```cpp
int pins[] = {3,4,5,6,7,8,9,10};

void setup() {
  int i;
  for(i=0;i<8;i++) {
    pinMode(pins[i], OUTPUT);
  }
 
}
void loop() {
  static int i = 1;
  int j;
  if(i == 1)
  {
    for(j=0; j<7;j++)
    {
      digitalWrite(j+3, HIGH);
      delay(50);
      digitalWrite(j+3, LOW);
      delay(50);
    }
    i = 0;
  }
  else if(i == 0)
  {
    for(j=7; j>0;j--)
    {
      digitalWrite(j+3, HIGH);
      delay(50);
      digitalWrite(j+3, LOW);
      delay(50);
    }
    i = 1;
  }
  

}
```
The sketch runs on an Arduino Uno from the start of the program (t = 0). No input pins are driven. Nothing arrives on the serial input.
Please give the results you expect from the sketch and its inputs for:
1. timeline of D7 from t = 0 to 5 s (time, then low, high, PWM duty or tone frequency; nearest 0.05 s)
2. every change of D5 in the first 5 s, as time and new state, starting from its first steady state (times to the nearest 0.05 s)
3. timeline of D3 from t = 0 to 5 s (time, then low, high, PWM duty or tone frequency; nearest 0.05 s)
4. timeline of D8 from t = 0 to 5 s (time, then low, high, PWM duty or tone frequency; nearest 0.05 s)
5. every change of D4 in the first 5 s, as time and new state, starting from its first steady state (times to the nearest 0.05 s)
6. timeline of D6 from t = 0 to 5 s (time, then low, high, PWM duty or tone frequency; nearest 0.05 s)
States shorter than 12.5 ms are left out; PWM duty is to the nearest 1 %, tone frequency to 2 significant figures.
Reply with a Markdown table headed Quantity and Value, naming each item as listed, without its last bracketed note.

| Quantity | Value |
|---|---|
| timeline of D7 from t = 0 to 5 s | 0 s low; 0.4 s high; 0.45 s low; 1 s high; 1.05 s low; 1.8 s high; 1.85 s low; 2.4 s high; 2.45 s low; 3.2 s high; 3.25 s low; 3.8 s high; 3.85 s low; 4.6 s high; 4.65 s low |
| every change of D5 in the first 5 s, as time and new state, starting from its first steady state | 0 s low; 0.2 s high; 0.25 s low; 1.2 s high; 1.25 s low; 1.6 s high; 1.65 s low; 2.6 s high; 2.65 s low; 3 s high; 3.05 s low; 4 s high; 4.05 s low; 4.4 s high; 4.45 s low |
| timeline of D3 from t = 0 to 5 s | 0 s high; 0.05 s low; 1.4 s high; 1.45 s low; 2.8 s high; 2.85 s low; 4.2 s high; 4.25 s low |
| timeline of D8 from t = 0 to 5 s | 0 s low; 0.5 s high; 0.55 s low; 0.9 s high; 0.95 s low; 1.9 s high; 1.95 s low; 2.3 s high; 2.35 s low; 3.3 s high; 3.35 s low; 3.7 s high; 3.75 s low; 4.7 s high; 4.75 s low |
| every change of D4 in the first 5 s, as time and new state, starting from its first steady state | 0 s low; 0.1 s high; 0.15 s low; 1.3 s high; 1.35 s low; 1.5 s high; 1.55 s low; 2.7 s high; 2.75 s low; 2.9 s high; 2.95 s low; 4.1 s high; 4.15 s low; 4.3 s high; 4.35 s low |
| timeline of D6 from t = 0 to 5 s | 0 s low; 0.3 s high; 0.35 s low; 1.1 s high; 1.15 s low; 1.7 s high; 1.75 s low; 2.5 s high; 2.55 s low; 3.1 s high; 3.15 s low; 3.9 s high; 3.95 s low; 4.5 s high; 4.55 s low |
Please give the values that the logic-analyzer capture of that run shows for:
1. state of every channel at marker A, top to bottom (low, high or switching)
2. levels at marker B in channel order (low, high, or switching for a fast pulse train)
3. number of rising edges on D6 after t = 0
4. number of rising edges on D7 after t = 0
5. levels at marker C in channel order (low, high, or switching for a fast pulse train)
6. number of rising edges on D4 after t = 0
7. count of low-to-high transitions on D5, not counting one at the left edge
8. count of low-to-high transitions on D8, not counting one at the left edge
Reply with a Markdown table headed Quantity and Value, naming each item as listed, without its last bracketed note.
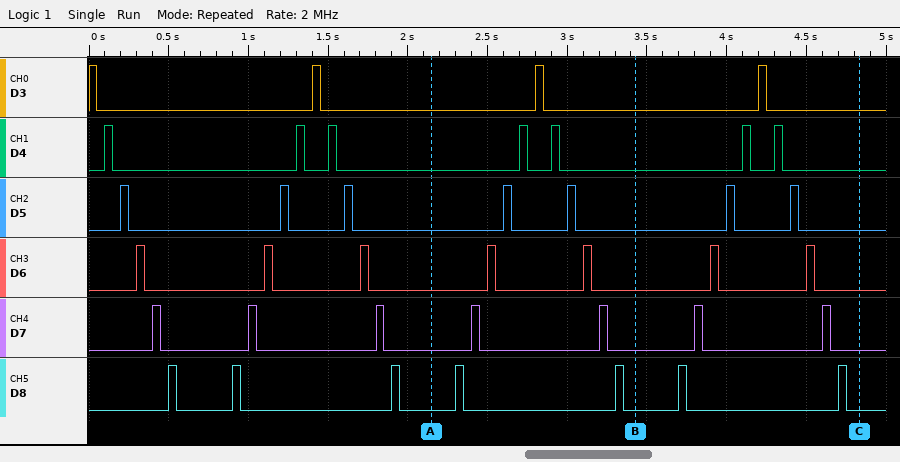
| Quantity | Value |
|---|---|
| state of every channel at marker A, top to bottom | D3 low, D4 low, D5 low, D6 low, D7 low, D8 low |
| levels at marker B in channel order | D3 low, D4 low, D5 low, D6 low, D7 low, D8 low |
| number of rising edges on D6 after t = 0 | 7 |
| number of rising edges on D7 after t = 0 | 7 |
| levels at marker C in channel order | D3 low, D4 low, D5 low, D6 low, D7 low, D8 low |
| number of rising edges on D4 after t = 0 | 7 |
| count of low-to-high transitions on D5, not counting one at the left edge | 7 |
| count of low-to-high transitions on D8, not counting one at the left edge | 7 |
